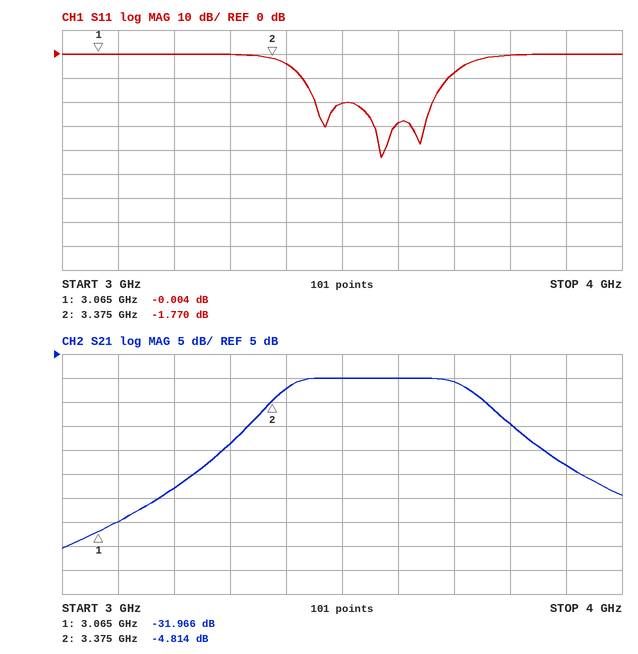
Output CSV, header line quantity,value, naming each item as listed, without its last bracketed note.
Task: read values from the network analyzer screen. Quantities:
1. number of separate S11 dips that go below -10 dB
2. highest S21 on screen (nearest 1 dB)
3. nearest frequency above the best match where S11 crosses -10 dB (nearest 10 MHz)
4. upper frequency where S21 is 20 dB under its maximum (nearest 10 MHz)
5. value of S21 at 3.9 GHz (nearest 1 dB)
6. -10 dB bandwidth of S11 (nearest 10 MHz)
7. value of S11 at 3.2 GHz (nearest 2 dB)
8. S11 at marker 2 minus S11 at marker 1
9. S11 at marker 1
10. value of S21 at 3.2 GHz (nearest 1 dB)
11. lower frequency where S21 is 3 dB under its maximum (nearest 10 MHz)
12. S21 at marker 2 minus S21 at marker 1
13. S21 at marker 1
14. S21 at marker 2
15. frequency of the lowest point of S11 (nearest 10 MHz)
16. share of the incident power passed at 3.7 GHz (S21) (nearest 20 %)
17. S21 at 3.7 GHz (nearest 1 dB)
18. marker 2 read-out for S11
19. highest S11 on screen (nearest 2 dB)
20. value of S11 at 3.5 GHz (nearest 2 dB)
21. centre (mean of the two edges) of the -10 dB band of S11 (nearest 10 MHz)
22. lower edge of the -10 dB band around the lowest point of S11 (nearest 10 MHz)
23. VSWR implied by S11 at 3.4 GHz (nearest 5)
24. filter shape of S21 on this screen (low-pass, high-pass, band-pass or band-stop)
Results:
quantity,value
number of separate S11 dips that go below -10 dB,3
highest S21 on screen,0 dB
nearest frequency above the best match where S11 crosses -10 dB,3.69 GHz
upper frequency where S21 is 20 dB under its maximum,3.93 GHz
value of S21 at 3.9 GHz,-18 dB
-10 dB bandwidth of S11,260 MHz
value of S11 at 3.2 GHz,0 dB
S11 at marker 2 minus S11 at marker 1,-1.766 dB
S11 at marker 1,-0.004 dB
value of S21 at 3.2 GHz,-23 dB
lower frequency where S21 is 3 dB under its maximum,3.39 GHz
S21 at marker 2 minus S21 at marker 1,27.152 dB
S21 at marker 1,-31.966 dB
S21 at marker 2,-4.814 dB
frequency of the lowest point of S11,3.57 GHz
share of the incident power passed at 3.7 GHz (S21),80 %
S21 at 3.7 GHz,-1 dB
marker 2 read-out for S11,-1.770 dB
highest S11 on screen,0 dB
value of S11 at 3.5 GHz,-20 dB
centre (mean of the two edges) of the -10 dB band of S11,3.56 GHz
lower edge of the -10 dB band around the lowest point of S11,3.43 GHz
VSWR implied by S11 at 3.4 GHz,5
filter shape of S21 on this screen,band-pass
